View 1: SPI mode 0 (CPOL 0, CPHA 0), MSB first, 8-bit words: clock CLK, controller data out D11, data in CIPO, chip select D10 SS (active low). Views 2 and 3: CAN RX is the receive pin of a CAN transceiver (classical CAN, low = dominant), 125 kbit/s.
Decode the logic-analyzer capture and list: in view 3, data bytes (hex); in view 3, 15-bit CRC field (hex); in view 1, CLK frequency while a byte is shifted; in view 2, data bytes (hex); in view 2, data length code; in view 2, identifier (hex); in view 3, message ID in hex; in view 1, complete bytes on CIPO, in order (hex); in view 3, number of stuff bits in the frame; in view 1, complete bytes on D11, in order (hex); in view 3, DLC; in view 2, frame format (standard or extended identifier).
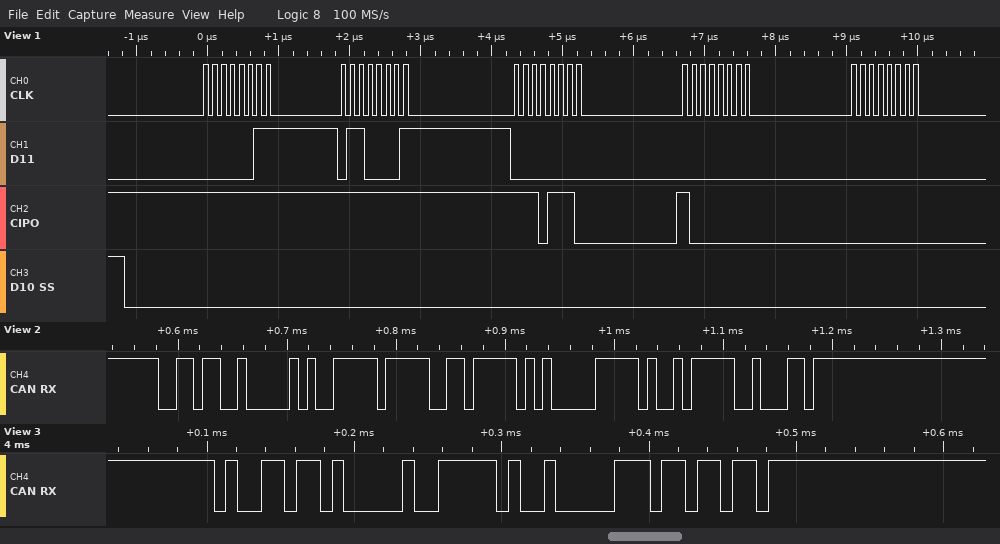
F9
0x036D
8 MHz
FF DB F4 1F
4
0x364
0x4DA
FF FF EE 80 00
3
03 61 00 00 00
1
standard
